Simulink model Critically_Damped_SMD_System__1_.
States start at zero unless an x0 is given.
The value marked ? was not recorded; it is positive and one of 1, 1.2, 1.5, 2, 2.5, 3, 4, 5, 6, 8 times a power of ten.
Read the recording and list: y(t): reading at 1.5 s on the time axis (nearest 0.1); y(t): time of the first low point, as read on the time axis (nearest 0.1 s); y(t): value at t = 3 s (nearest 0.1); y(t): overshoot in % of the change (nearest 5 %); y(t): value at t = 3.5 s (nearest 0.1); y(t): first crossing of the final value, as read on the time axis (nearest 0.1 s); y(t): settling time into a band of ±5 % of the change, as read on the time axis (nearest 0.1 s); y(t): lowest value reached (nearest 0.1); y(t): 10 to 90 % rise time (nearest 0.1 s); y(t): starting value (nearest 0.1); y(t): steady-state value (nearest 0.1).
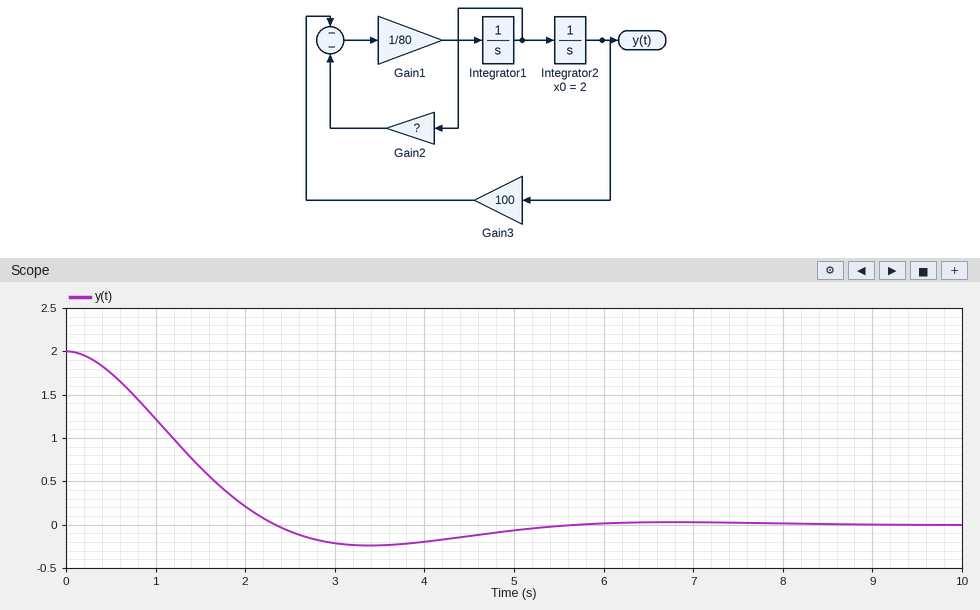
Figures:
0.7
3.4 s
-0.2
10 %
-0.2
2.3 s
4.7 s
-0.2
1.6 s
2.0
0.0
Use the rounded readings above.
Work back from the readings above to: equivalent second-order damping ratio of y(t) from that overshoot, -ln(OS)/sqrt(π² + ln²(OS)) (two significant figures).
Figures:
0.59
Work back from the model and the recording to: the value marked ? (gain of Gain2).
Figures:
100
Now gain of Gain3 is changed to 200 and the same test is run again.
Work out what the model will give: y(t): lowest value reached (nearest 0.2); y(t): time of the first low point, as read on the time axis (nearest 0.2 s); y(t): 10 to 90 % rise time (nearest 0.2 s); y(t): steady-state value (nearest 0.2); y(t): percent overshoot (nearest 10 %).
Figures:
-0.6
2.2 s
1.0 s
0.0
30 %
